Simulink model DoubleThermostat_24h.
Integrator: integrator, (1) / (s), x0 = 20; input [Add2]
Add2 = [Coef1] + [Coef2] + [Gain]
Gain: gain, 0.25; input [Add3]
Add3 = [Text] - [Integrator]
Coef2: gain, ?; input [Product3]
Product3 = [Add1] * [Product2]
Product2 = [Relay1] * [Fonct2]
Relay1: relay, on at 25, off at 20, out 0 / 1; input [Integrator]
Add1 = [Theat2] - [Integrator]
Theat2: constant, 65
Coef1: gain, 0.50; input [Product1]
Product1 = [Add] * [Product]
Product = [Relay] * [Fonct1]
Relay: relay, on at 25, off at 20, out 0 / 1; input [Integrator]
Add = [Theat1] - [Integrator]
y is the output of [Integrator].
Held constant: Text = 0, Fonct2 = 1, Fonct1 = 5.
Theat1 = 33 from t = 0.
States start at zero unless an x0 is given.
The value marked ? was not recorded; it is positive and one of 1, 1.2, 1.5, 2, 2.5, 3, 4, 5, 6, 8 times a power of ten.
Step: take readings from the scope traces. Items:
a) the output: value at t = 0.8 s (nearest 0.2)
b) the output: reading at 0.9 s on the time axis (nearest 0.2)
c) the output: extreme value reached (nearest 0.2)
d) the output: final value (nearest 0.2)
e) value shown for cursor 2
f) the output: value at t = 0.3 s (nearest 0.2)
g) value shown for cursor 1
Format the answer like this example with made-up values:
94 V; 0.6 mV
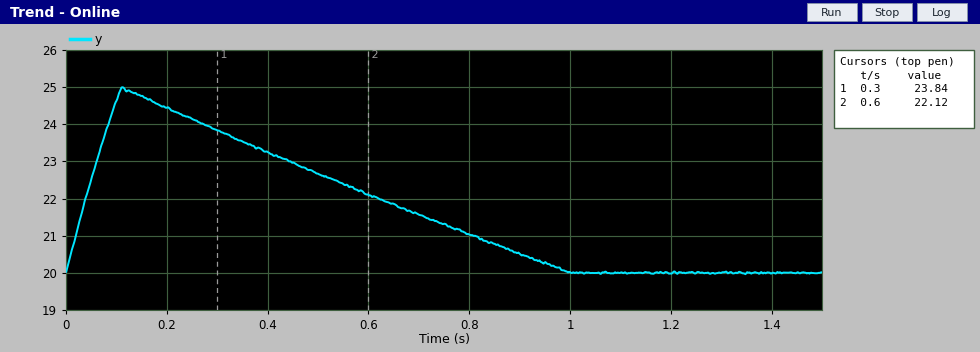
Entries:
21.0; 20.6; 25.0; 20.0; 22.12; 23.8; 23.84
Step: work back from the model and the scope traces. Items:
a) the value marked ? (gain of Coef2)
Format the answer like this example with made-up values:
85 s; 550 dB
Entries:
0.6
